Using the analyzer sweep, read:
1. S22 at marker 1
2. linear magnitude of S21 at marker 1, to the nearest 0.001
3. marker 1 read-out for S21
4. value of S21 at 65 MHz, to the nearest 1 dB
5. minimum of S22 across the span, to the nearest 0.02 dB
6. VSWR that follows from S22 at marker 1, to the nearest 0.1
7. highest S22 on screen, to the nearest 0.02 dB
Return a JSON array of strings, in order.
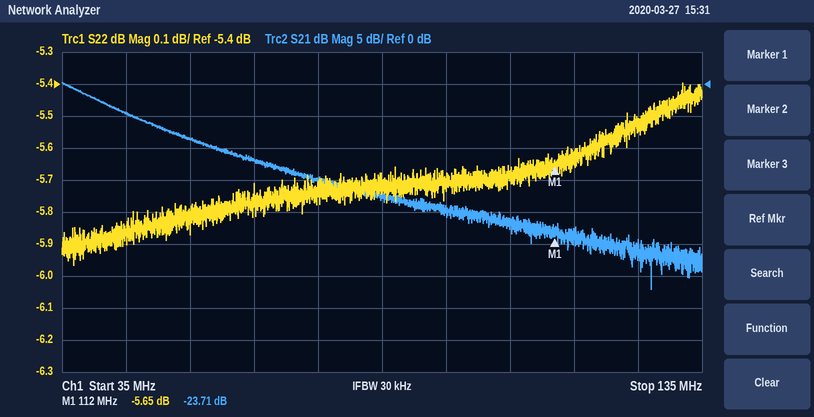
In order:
["-5.65 dB", "0.065", "-23.71 dB", "-12 dB", "-5.96 dB", "3.2", "-5.40 dB"]
